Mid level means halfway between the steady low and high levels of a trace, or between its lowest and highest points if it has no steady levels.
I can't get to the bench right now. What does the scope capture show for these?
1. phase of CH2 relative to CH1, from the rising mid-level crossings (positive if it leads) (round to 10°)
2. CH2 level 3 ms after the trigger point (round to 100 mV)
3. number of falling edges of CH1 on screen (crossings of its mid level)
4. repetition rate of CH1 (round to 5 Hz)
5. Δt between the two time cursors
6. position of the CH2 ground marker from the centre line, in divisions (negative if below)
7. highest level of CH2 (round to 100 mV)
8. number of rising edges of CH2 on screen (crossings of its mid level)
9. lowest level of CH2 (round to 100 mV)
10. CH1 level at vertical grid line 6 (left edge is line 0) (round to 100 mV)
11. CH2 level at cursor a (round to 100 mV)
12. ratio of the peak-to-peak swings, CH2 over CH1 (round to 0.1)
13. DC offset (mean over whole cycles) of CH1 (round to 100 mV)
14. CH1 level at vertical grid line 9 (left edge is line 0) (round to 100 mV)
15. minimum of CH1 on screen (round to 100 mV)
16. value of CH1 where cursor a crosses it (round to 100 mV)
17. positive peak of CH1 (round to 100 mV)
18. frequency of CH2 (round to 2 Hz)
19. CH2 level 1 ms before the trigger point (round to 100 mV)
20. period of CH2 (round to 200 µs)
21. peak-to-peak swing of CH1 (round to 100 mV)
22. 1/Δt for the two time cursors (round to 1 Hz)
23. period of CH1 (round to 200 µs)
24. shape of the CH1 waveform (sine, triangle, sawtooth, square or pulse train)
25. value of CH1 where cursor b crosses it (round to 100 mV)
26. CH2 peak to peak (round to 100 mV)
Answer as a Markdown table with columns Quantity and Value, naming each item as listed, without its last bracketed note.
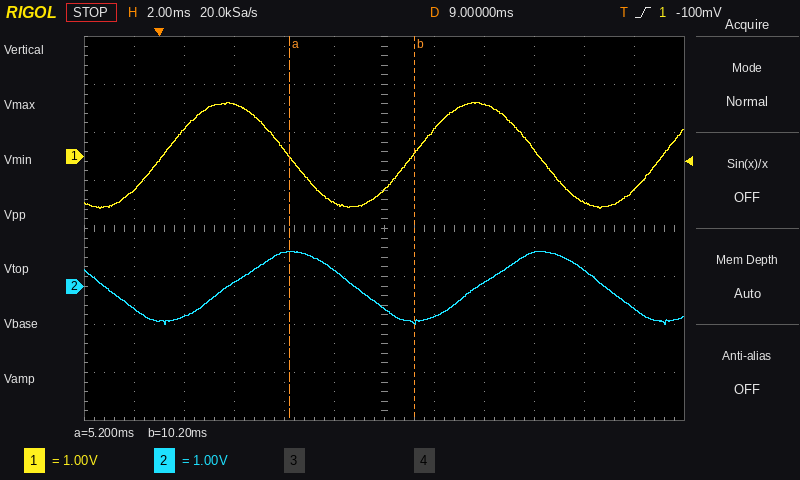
| Quantity | Value |
|---|---|
| phase of CH2 relative to CH1, from the rising mid-level crossings (positive if it leads) | -90° |
| CH2 level 3 ms after the trigger point | 100 mV |
| number of falling edges of CH1 on screen | 2 |
| repetition rate of CH1 | 100 Hz |
| Δt between the two time cursors | 5.0 ms |
| position of the CH2 ground marker from the centre line, in divisions | -1.2 div |
| highest level of CH2 | 700 mV |
| number of rising edges of CH2 on screen | 2 |
| lowest level of CH2 | -800 mV |
| CH1 level at vertical grid line 6 (left edge is line 0) | -700 mV |
| CH2 level at cursor a | 700 mV |
| ratio of the peak-to-peak swings, CH2 over CH1 | 0.7 |
| DC offset (mean over whole cycles) of CH1 | 0.0 V |
| CH1 level at vertical grid line 9 (left edge is line 0) | 100 mV |
| minimum of CH1 on screen | -1.1 V |
| value of CH1 where cursor a crosses it | 0.0 V |
| positive peak of CH1 | 1.1 V |
| frequency of CH2 | 100 Hz |
| CH2 level 1 ms before the trigger point | -500 mV |
| period of CH2 | 10.0 ms |
| peak-to-peak swing of CH1 | 2.2 V |
| 1/Δt for the two time cursors | 200 Hz |
| period of CH1 | 10.0 ms |
| shape of the CH1 waveform | sine |
| value of CH1 where cursor b crosses it | 100 mV |
| CH2 peak to peak | 1.5 V |
